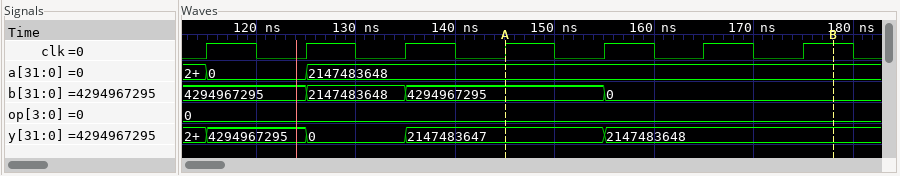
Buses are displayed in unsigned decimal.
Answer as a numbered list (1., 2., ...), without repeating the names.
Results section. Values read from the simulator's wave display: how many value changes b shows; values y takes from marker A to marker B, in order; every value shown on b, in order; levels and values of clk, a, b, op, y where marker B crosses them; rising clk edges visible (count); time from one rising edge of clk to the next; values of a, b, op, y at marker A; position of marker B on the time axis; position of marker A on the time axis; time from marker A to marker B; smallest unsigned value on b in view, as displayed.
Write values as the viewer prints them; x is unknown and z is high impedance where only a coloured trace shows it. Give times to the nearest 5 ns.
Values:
1. 3
2. 2147483647, 2147483648
3. 4294967295, 2147483648, 4294967295, 0
4. clk=1, a=2147483648, b=0, op=0, y=2147483648
5. 7
6. 10 ns
7. a=2147483648, b=4294967295, op=0, y=2147483647
8. 180 ns
9. 145 ns
10. 35 ns
11. 0
